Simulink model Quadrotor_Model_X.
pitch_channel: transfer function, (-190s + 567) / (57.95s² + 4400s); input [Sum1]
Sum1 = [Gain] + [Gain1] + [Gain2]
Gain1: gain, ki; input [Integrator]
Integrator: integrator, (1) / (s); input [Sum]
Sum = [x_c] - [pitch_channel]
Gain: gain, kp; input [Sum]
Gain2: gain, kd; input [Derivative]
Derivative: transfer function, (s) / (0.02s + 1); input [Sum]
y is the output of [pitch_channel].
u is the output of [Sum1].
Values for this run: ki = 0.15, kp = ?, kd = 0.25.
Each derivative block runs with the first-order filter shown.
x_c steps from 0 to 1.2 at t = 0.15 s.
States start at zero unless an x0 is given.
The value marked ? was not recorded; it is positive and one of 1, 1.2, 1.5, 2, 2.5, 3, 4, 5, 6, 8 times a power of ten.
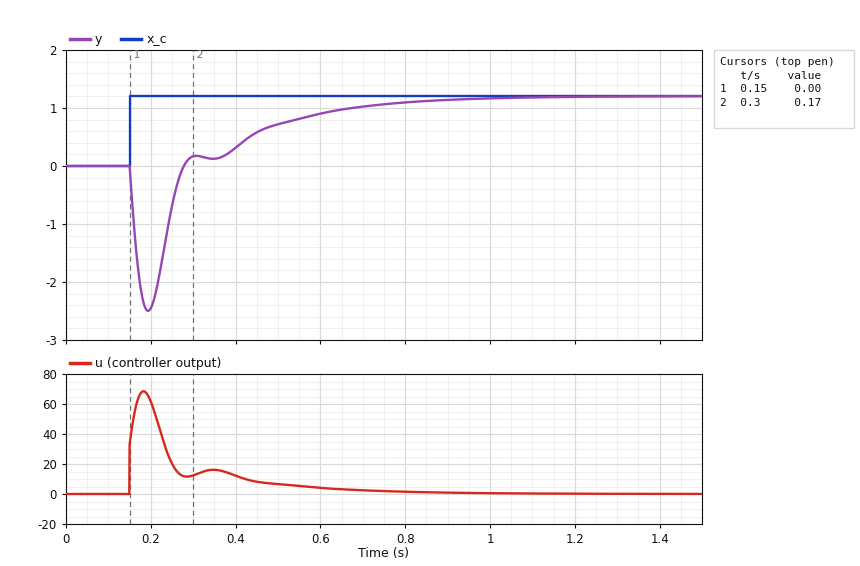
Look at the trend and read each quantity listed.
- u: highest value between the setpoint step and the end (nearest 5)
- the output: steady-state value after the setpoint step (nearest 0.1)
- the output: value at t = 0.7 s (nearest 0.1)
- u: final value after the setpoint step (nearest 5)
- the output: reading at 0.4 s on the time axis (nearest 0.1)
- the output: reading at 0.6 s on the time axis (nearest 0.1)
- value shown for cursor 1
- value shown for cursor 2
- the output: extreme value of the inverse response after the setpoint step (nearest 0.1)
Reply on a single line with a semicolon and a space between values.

70; 1.2; 1.0; 0; 0.3; 0.9; 0.00; 0.17; -2.5
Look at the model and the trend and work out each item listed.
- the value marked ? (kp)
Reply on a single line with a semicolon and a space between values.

15
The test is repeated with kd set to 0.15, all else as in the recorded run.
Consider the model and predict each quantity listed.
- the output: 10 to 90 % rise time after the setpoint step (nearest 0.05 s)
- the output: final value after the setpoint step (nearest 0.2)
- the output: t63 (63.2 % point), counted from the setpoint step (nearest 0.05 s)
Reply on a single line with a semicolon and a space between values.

0.40 s; 1.2; 0.35 s
